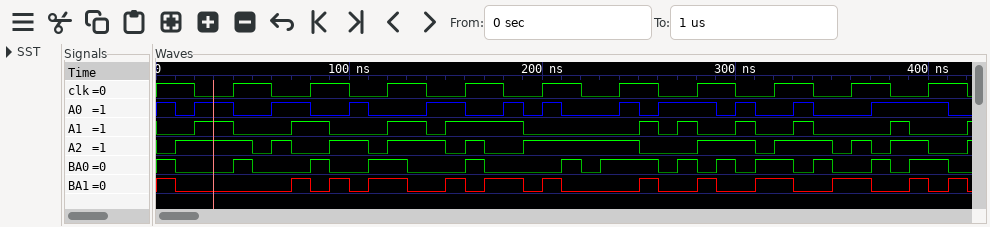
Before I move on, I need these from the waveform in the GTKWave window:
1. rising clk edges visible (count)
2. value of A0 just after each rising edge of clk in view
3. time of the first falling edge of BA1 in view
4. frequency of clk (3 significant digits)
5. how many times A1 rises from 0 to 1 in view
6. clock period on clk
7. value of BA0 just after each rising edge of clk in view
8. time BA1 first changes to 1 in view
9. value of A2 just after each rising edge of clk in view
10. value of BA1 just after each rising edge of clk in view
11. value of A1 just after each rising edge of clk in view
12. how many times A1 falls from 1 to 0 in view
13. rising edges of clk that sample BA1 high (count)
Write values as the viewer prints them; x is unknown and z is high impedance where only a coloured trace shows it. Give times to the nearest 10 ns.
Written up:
10
0 0 0 0 1 1 1 0 0 1
10 ns
25.0 MHz
10
40 ns
1 1 1 1 0 1 0 1 0 1
70 ns
1 0 1 1 1 1 1 1 1 0
0 0 1 0 1 0 1 1 1 0
0 1 1 1 0 0 0 0 0 0
9
6
